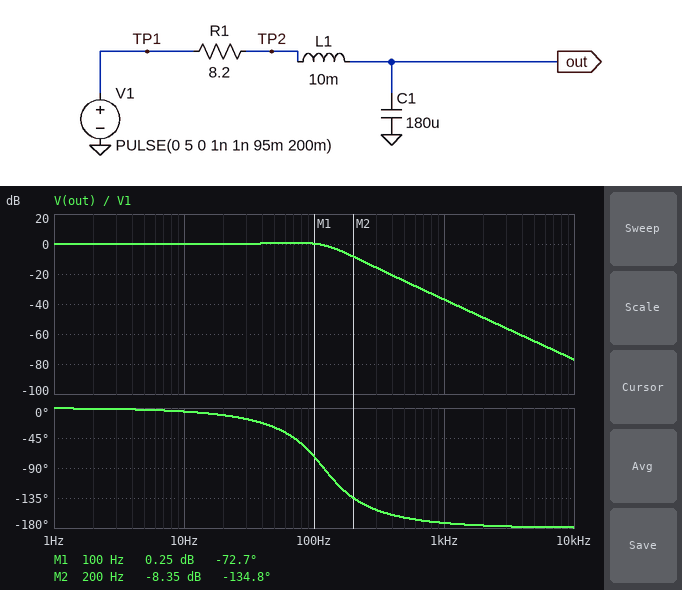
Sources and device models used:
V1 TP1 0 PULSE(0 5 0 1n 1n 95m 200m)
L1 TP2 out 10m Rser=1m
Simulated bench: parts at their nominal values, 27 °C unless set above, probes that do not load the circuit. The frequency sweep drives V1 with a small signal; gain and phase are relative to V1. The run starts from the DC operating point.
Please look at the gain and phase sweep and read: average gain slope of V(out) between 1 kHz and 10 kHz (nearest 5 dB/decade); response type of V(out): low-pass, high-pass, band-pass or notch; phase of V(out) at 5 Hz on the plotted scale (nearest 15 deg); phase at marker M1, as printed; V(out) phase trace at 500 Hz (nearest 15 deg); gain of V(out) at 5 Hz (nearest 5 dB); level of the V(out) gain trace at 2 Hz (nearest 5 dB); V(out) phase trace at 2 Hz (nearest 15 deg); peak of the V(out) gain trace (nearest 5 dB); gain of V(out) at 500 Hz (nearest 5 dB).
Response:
-40 dB/decade
low-pass
0 deg
-72.7 deg
-165 deg
0 dB
0 dB
0 deg
0 dB
-25 dB
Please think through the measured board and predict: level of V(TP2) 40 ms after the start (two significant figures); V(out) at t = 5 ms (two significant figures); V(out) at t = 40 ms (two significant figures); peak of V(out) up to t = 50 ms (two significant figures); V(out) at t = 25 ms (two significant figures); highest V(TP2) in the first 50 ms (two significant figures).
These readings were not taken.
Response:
5.0 V
5.6 V
5.0 V
5.6 V
5.0 V
5.4 V
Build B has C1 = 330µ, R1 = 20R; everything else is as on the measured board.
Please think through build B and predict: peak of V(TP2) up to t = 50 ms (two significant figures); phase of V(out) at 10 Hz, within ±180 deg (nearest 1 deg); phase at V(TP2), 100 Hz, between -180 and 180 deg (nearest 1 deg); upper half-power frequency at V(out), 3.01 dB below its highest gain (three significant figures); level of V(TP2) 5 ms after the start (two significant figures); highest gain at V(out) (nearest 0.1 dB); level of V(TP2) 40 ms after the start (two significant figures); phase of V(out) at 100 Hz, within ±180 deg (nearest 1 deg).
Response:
5.0 V
-23 deg
86 deg
26.1 Hz
2.4 V
0 dB
5.0 V
-94 deg
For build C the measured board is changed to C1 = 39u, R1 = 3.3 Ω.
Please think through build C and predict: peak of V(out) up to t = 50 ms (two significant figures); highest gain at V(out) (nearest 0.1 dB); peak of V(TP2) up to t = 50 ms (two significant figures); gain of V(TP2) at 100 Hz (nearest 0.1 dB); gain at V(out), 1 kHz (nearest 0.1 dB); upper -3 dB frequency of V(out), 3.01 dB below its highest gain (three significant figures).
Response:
8.6 V
13.8 dB
5.6 V
0 dB
-23.2 dB
277 Hz
